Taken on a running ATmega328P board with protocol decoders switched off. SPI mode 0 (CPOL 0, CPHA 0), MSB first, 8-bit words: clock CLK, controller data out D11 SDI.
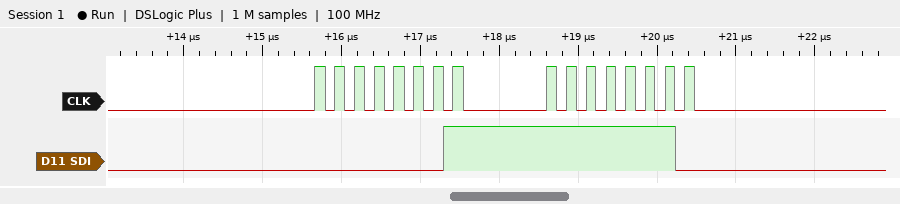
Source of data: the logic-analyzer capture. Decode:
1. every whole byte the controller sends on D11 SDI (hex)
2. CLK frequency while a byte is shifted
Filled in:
01 FE
4 MHz
